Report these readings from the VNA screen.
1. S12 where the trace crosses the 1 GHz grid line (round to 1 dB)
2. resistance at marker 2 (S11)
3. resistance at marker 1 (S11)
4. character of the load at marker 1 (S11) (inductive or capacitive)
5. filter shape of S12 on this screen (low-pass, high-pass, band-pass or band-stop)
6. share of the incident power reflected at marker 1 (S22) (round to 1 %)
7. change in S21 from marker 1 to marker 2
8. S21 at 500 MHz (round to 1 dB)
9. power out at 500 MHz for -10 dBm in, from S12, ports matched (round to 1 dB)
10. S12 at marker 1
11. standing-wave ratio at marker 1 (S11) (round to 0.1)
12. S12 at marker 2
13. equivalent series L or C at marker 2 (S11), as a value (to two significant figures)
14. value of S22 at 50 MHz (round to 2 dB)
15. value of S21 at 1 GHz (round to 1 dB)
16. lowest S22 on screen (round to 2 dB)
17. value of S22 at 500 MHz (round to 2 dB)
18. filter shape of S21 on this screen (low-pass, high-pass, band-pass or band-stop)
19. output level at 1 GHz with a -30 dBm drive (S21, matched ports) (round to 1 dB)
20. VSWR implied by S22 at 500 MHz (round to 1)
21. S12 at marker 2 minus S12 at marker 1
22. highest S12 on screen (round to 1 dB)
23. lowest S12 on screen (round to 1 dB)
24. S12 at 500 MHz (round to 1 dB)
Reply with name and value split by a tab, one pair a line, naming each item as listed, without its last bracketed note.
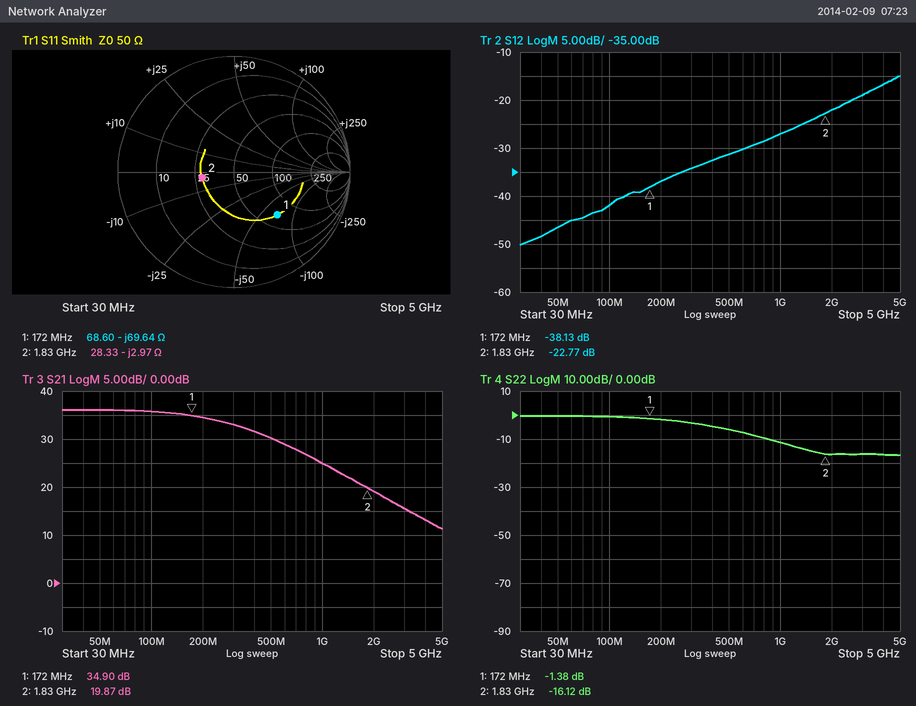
S12 where the trace crosses the 1 GHz grid line	-27 dB
resistance at marker 2	28.33 Ω
resistance at marker 1	68.60 Ω
character of the load at marker 1 (S11)	capacitive
filter shape of S12 on this screen	high-pass
share of the incident power reflected at marker 1 (S22)	73 %
change in S21 from marker 1 to marker 2	-15.03 dB
S21 at 500 MHz	30 dB
power out at 500 MHz for -10 dBm in, from S12, ports matched	-41 dBm
S12 at marker 1	-38.13 dB
standing-wave ratio at marker 1 (S11)	3.2
S12 at marker 2	-22.77 dB
equivalent series L or C at marker 2 (S11), as a value	29 pF
value of S22 at 50 MHz	0 dB
value of S21 at 1 GHz	25 dB
lowest S22 on screen	-16 dB
value of S22 at 500 MHz	-6 dB
filter shape of S21 on this screen	low-pass
output level at 1 GHz with a -30 dBm drive (S21, matched ports)	-5 dBm
VSWR implied by S22 at 500 MHz	3
S12 at marker 2 minus S12 at marker 1	15.36 dB
highest S12 on screen	-15 dB
lowest S12 on screen	-50 dB
S12 at 500 MHz	-31 dB
